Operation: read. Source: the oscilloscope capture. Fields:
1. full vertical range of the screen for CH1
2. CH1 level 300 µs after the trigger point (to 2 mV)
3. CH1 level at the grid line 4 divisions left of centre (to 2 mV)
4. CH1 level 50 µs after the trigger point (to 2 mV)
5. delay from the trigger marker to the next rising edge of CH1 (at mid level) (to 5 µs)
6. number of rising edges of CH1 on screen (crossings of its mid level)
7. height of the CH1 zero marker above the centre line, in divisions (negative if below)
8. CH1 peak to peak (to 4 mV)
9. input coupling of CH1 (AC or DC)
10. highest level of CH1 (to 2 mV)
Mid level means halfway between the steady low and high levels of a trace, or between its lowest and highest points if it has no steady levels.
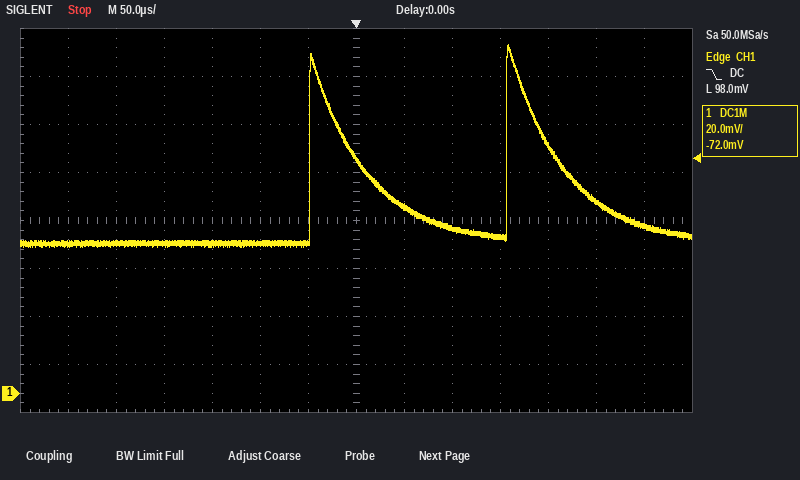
160 mV
70 mV
62 mV
78 mV
155 µs
2
-3.6 div
84 mV
DC
146 mV
